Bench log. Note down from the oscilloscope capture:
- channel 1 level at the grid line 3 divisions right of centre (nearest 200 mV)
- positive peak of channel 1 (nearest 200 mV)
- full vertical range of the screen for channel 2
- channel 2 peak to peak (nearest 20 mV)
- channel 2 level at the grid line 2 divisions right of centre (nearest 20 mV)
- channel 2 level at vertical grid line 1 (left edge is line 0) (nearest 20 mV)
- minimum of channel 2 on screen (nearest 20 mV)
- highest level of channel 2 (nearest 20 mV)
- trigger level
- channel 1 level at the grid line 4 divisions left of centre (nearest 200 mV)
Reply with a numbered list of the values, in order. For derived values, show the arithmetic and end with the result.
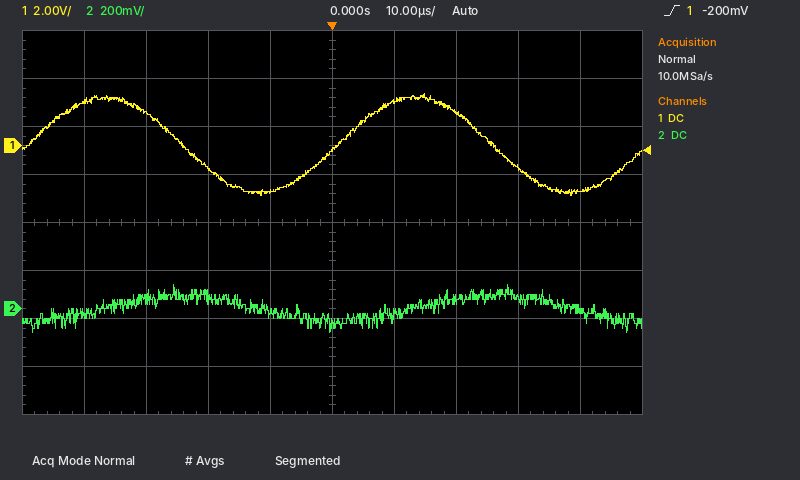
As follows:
1. -1.0 V
2. 2.2 V
3. 1.6 V
4. 100 mV − (-100 mV) = 200 mV
5. 40 mV
6. -20 mV
7. -100 mV
8. 100 mV
9. -200 mV
10. 1.8 V
